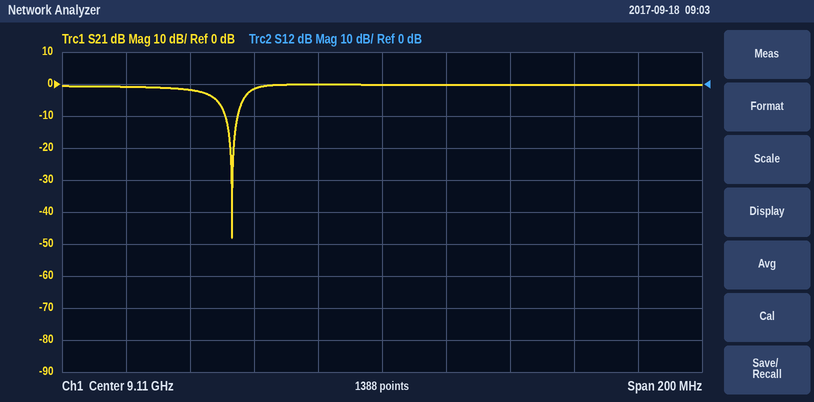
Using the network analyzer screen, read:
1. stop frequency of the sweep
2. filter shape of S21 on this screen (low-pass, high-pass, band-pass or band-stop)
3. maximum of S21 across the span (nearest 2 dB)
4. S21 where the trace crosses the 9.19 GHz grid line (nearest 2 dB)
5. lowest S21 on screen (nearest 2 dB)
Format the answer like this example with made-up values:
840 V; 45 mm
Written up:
9.21 GHz; band-stop; 0 dB; 0 dB; -48 dB
